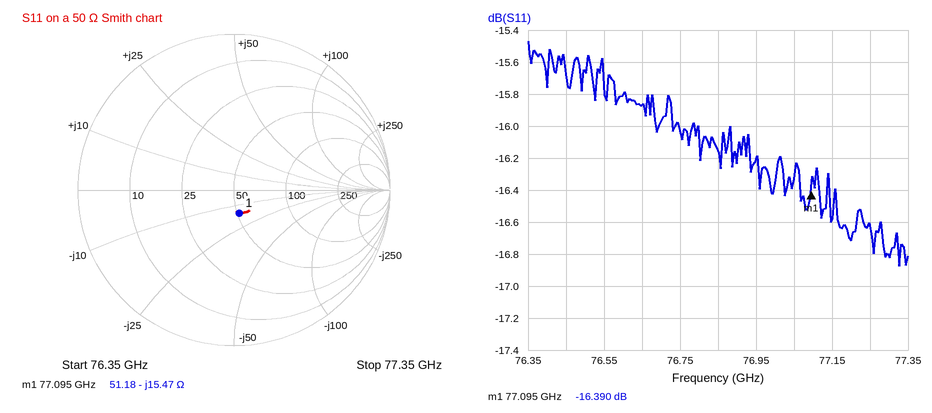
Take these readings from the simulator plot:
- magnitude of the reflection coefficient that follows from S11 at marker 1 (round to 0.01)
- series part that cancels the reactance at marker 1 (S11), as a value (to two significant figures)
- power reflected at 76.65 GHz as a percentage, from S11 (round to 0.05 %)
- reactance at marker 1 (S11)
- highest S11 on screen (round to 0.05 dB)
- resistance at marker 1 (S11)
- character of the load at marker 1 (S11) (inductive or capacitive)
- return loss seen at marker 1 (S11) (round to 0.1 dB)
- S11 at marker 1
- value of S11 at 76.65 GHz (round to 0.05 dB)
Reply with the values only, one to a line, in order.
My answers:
0.15
32 pH
2.60 %
-15.47 Ω
-15.45 dB
51.18 Ω
capacitive
16.4 dB
-16.390 dB
-15.85 dB
